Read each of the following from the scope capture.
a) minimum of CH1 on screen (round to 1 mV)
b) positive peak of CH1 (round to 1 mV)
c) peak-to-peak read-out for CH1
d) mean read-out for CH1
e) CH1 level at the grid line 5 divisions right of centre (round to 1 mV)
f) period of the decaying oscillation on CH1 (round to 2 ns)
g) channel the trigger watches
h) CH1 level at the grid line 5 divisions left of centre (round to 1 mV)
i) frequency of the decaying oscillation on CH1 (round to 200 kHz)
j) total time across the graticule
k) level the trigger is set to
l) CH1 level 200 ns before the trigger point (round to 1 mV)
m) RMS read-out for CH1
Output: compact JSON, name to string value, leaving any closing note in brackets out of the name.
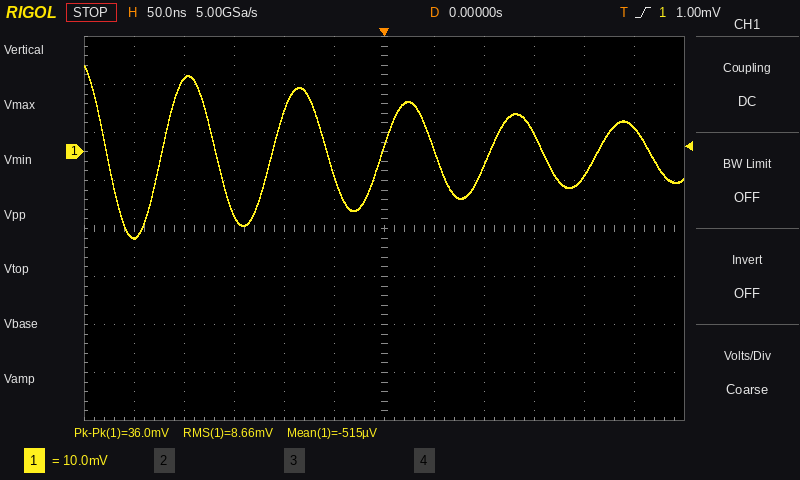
{"minimum of CH1 on screen": "-18 mV", "positive peak of CH1": "18 mV", "peak-to-peak read-out for CH1": "36.0 mV", "mean read-out for CH1": "-515 µV", "CH1 level at the grid line 5 divisions right of centre": "5 mV", "period of the decaying oscillation on CH1": "108 ns", "channel the trigger watches": "CH1", "CH1 level at the grid line 5 divisions left of centre": "-18 mV", "frequency of the decaying oscillation on CH1": "9.2 MHz", "total time across the graticule": "600 ns", "level the trigger is set to": "1.00 mV", "CH1 level 200 ns before the trigger point": "15 mV", "RMS read-out for CH1": "8.66 mV"}
